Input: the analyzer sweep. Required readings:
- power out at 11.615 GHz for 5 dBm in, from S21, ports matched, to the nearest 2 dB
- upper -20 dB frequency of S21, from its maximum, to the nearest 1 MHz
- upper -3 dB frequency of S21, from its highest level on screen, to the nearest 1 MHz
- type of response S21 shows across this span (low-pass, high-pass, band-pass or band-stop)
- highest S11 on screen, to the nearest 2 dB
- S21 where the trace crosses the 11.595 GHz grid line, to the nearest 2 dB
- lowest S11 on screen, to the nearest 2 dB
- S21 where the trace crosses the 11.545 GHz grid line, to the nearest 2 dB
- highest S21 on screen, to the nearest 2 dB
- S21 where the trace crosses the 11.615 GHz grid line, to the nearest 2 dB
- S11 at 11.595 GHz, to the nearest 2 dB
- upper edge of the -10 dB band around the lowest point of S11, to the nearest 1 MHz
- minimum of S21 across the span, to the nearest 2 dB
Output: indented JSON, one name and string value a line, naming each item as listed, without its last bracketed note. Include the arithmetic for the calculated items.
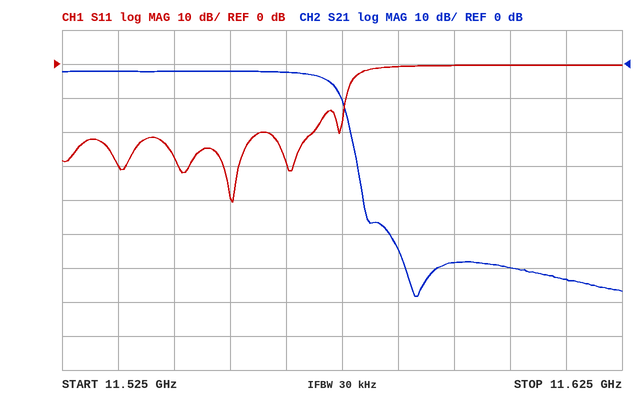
{
  "power out at 11.615 GHz for 5 dBm in, from S21, ports matched, to the nearest 2 dB": "5 dBm + (-64 dB) = -58 dBm",
  "upper -20 dB frequency of S21, from its maximum, to the nearest 1 MHz": "11.577 GHz",
  "upper -3 dB frequency of S21, from its highest level on screen, to the nearest 1 MHz": "11.573 GHz",
  "type of response S21 shows across this span": "low-pass",
  "highest S11 on screen, to the nearest 2 dB": "0 dB",
  "S21 where the trace crosses the 11.595 GHz grid line, to the nearest 2 dB": "-58 dB",
  "lowest S11 on screen, to the nearest 2 dB": "-40 dB",
  "S21 where the trace crosses the 11.545 GHz grid line, to the nearest 2 dB": "-2 dB",
  "highest S21 on screen, to the nearest 2 dB": "-2 dB",
  "S21 where the trace crosses the 11.615 GHz grid line, to the nearest 2 dB": "-64 dB",
  "S11 at 11.595 GHz, to the nearest 2 dB": "0 dB",
  "upper edge of the -10 dB band around the lowest point of S11, to the nearest 1 MHz": "11.576 GHz",
  "minimum of S21 across the span, to the nearest 2 dB": "-68 dB"
}
